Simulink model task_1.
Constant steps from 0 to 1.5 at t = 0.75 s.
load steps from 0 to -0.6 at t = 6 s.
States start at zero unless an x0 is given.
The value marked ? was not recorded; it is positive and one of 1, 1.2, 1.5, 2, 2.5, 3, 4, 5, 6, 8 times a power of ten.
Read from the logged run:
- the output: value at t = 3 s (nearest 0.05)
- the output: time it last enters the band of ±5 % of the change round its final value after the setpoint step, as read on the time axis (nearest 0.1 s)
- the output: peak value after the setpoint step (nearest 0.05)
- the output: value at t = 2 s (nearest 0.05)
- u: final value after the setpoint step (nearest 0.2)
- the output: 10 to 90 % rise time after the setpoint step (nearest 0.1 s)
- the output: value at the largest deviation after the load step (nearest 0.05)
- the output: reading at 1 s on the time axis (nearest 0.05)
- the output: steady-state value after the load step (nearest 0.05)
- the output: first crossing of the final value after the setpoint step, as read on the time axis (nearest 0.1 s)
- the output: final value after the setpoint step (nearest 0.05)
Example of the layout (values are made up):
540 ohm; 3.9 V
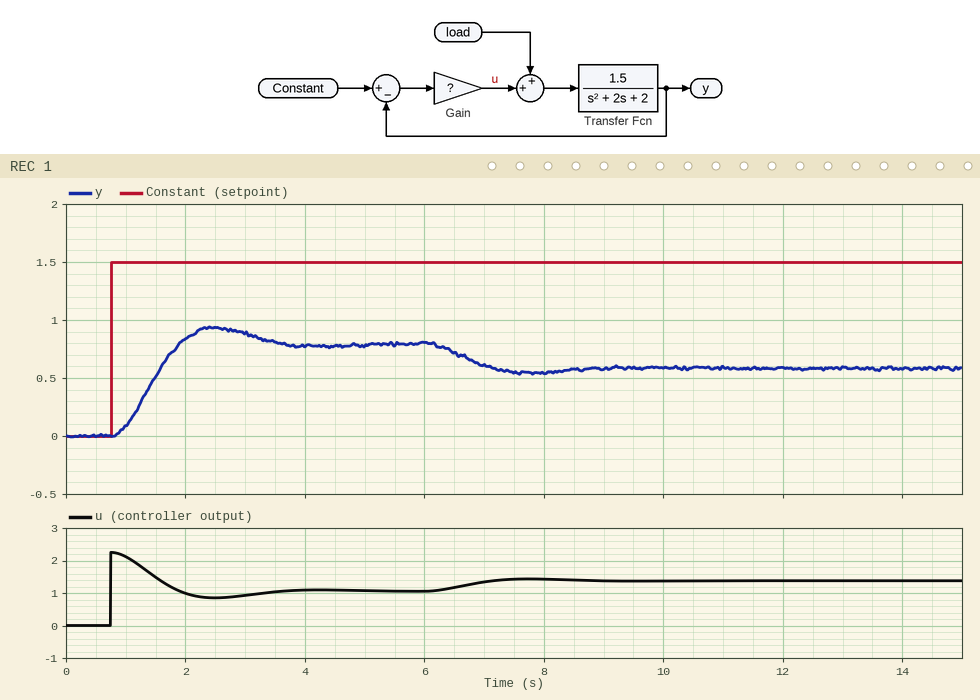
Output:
0.90; 3.3 s; 0.95; 0.85; 1.0; 0.8 s; 0.55; 0.10; 0.60; 1.9 s; 0.80
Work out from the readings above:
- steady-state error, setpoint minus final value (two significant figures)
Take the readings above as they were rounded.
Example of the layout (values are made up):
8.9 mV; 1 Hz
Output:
0.70
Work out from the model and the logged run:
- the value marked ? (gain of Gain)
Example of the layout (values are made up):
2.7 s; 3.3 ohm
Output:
1.5
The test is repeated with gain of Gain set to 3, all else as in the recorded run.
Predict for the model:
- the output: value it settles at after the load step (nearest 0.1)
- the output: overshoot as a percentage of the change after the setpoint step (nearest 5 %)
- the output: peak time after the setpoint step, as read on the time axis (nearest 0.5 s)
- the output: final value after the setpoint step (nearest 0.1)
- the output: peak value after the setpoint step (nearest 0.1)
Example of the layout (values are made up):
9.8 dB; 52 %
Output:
0.9; 25 %; 2.0 s; 1.0; 1.3
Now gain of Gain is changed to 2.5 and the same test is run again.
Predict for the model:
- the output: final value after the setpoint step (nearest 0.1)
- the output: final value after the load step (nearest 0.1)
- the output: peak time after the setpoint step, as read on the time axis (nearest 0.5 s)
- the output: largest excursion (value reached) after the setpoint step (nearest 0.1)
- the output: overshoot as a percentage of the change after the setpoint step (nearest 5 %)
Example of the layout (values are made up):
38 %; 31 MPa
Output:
1.0; 0.8; 2.0 s; 1.2; 25 %
